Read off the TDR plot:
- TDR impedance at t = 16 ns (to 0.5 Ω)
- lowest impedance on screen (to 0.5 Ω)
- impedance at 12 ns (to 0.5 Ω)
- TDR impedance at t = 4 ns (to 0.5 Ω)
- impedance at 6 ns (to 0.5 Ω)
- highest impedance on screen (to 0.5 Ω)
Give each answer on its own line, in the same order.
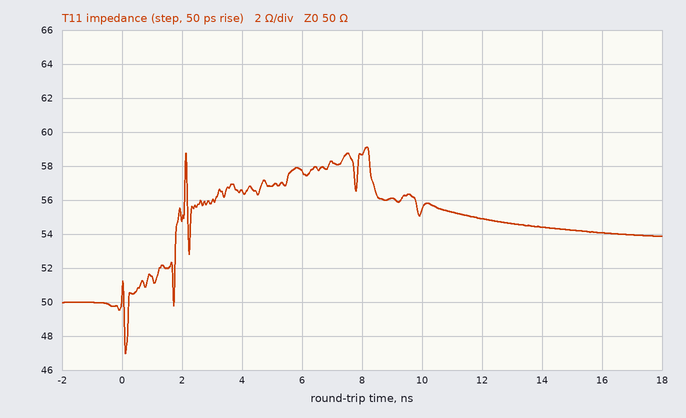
54.0 Ω
47.0 Ω
55.0 Ω
56.5 Ω
57.5 Ω
59.0 Ω
